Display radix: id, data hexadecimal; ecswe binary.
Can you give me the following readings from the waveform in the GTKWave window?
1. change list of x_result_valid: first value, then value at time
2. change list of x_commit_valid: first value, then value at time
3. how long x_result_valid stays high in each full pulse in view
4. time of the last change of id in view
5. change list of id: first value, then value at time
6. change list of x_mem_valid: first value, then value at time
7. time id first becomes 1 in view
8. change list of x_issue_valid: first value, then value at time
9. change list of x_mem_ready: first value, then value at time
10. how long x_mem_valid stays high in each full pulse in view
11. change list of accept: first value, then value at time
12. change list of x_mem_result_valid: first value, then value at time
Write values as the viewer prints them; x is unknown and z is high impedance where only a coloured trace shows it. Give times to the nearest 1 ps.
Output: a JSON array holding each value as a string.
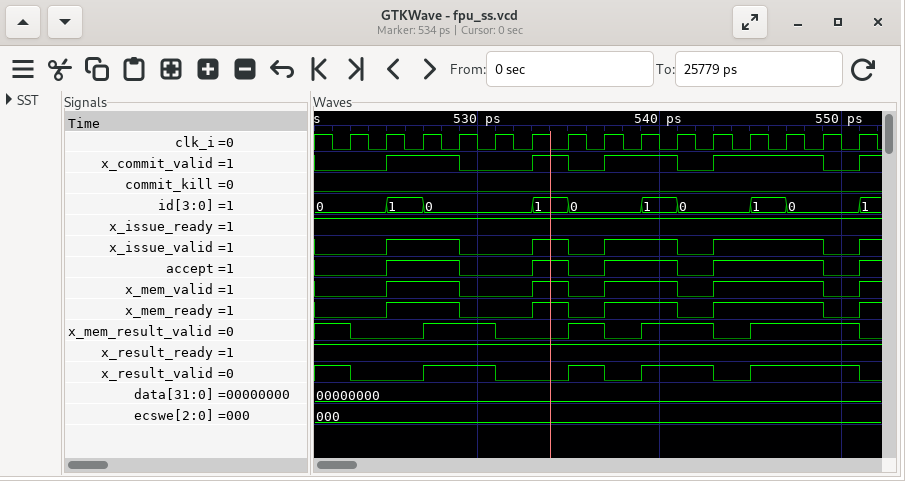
["1, 0 at 523 ps, 1 at 527 ps, 0 at 531 ps, 1 at 535 ps, 0 at 537 ps, 1 at 539 ps, 0 at 543 ps, 1 at 545 ps, 0 at 551 ps", "0, 1 at 525 ps, 0 at 529 ps, 1 at 533 ps, 0 at 535 ps, 1 at 537 ps, 0 at 541 ps, 1 at 543 ps, 0 at 549 ps, 1 at 551 ps", "4 ps, 2 ps, 4 ps, 6 ps", "551 ps", "0, 1 at 525 ps, 0 at 527 ps, 1 at 533 ps, 0 at 535 ps, 1 at 539 ps, 0 at 541 ps, 1 at 545 ps, 0 at 547 ps, 1 at 551 ps", "0, 1 at 525 ps, 0 at 529 ps, 1 at 533 ps, 0 at 535 ps, 1 at 537 ps, 0 at 541 ps, 1 at 543 ps, 0 at 549 ps, 1 at 551 ps", "525 ps", "0, 1 at 525 ps, 0 at 529 ps, 1 at 533 ps, 0 at 535 ps, 1 at 537 ps, 0 at 541 ps, 1 at 543 ps, 0 at 549 ps, 1 at 551 ps", "0, 1 at 525 ps, 0 at 529 ps, 1 at 533 ps, 0 at 535 ps, 1 at 537 ps, 0 at 541 ps, 1 at 543 ps, 0 at 549 ps, 1 at 551 ps", "4 ps, 2 ps, 4 ps, 6 ps", "0, 1 at 525 ps, 0 at 529 ps, 1 at 533 ps, 0 at 535 ps, 1 at 537 ps, 0 at 541 ps, 1 at 543 ps, 0 at 549 ps, 1 at 551 ps", "1, 0 at 523 ps, 1 at 527 ps, 0 at 531 ps, 1 at 535 ps, 0 at 537 ps, 1 at 539 ps, 0 at 543 ps, 1 at 545 ps, 0 at 551 ps"]
